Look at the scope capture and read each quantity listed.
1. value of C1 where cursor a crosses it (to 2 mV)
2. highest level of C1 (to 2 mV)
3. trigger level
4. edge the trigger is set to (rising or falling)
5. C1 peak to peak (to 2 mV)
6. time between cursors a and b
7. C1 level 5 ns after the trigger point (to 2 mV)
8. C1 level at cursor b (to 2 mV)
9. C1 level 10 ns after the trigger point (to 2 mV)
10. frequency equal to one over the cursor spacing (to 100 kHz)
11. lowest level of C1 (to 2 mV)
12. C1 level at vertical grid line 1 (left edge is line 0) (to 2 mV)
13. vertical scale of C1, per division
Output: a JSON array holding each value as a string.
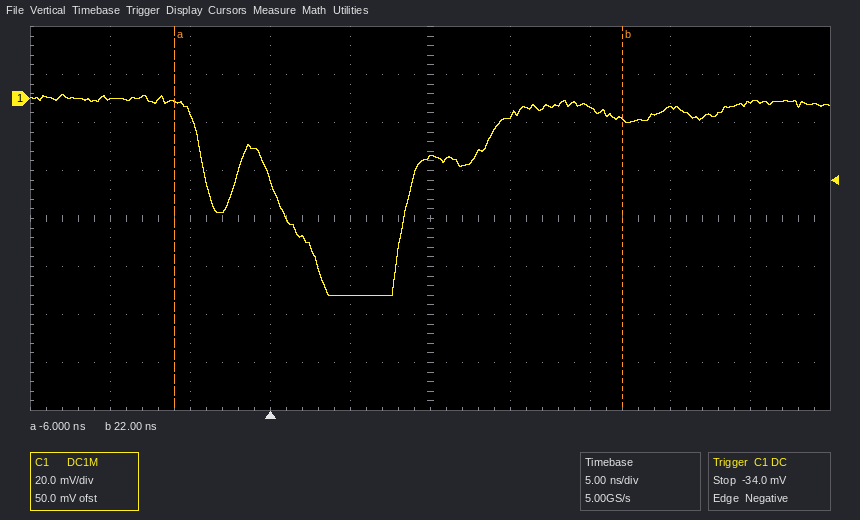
["-2 mV", "2 mV", "-34.0 mV", "falling", "84 mV", "28.0 ns", "-82 mV", "-8 mV", "-24 mV", "35.7 MHz", "-82 mV", "0 mV", "20 mV"]
